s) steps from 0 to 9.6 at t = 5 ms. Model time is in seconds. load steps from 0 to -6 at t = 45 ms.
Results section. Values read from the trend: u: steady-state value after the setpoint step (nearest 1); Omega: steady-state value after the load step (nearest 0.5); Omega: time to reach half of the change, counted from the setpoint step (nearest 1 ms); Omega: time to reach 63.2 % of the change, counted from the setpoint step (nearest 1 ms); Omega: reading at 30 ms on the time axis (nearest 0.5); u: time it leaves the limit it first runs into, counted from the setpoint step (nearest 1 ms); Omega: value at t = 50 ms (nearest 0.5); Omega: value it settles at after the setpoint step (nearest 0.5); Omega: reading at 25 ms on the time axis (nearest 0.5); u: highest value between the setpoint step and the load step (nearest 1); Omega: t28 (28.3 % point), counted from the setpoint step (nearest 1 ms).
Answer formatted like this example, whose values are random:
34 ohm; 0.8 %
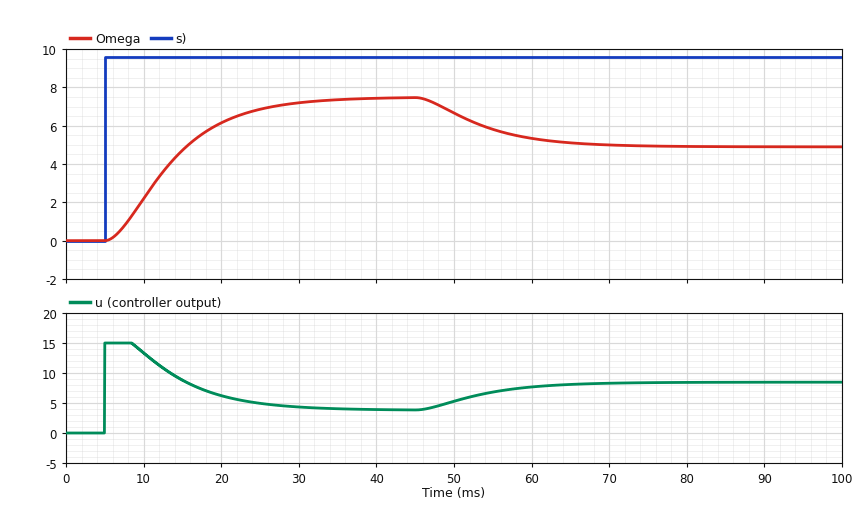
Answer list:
4; 5.0; 8 ms; 10 ms; 7.0; 4 ms; 6.5; 7.5; 7.0; 15; 5 ms
